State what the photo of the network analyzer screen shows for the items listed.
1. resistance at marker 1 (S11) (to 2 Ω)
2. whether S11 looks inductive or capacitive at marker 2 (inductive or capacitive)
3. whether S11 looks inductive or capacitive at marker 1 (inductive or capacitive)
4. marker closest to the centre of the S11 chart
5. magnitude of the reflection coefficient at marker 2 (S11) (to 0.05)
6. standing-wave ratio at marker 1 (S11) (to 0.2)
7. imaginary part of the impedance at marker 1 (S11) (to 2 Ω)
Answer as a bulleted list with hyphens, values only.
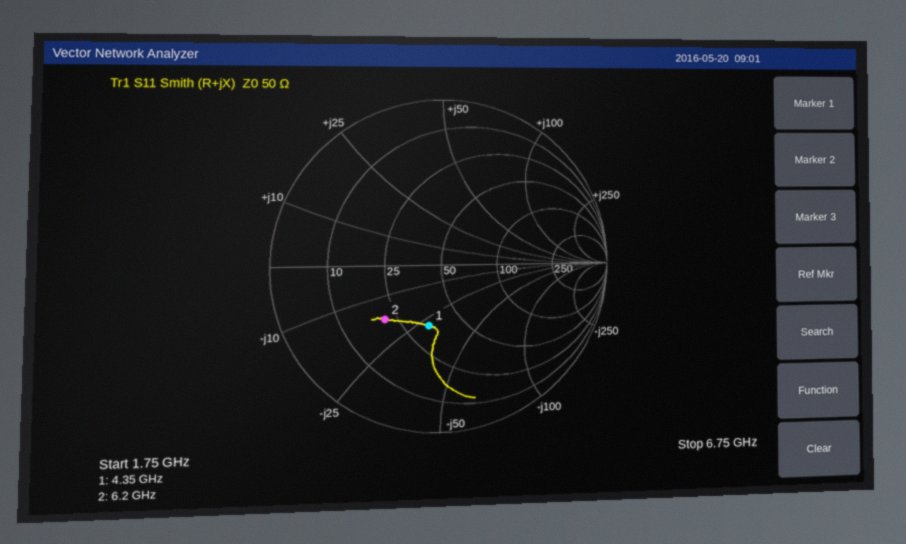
- 34 Ω
- capacitive
- capacitive
- marker 1
- 0.45
- 2.2
- -28 Ω
